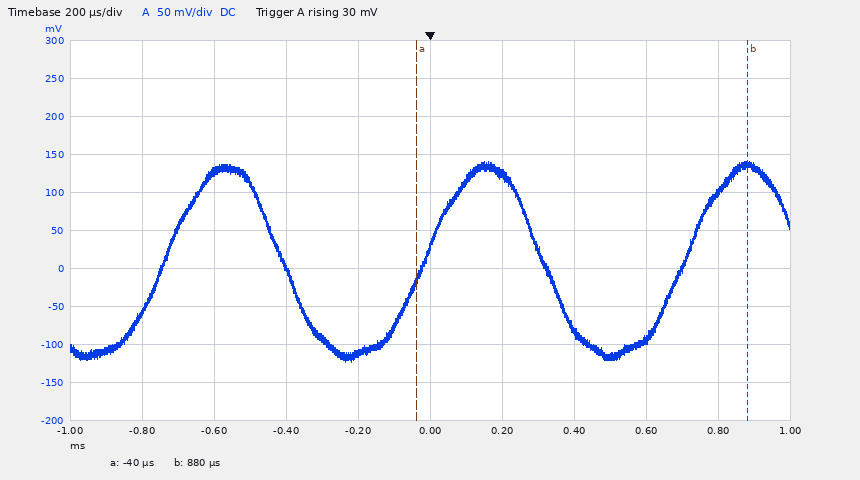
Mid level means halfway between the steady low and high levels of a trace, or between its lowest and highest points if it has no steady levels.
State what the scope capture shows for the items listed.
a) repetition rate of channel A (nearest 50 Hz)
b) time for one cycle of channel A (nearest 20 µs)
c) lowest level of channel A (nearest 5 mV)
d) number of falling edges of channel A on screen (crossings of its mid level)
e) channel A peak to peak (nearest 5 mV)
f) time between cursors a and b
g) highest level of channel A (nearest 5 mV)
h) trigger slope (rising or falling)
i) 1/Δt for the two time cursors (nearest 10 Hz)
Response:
1.40 kHz
720 µs
-125 mV
2
265 mV
920 µs
140 mV
rising
1.09 kHz
